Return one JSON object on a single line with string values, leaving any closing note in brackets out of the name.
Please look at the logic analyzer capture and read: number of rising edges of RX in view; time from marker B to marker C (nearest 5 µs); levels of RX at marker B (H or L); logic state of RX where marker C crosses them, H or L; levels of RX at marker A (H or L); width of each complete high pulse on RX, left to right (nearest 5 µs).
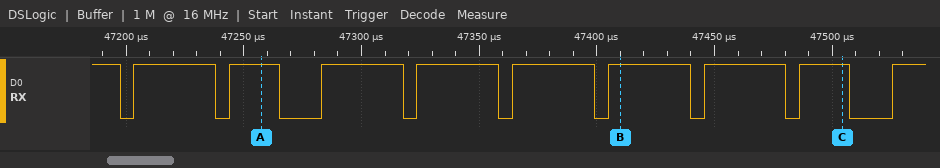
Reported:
{"number of rising edges of RX in view": "9", "time from marker B to marker C": "95 µs", "levels of RX at marker B": "RX=H", "logic state of RX where marker C crosses them, H or L": "RX=H", "levels of RX at marker A": "RX=H", "width of each complete high pulse on RX, left to right": "35 µs, 20 µs, 35 µs, 35 µs, 35 µs, 35 µs, 35 µs, 20 µs"}
